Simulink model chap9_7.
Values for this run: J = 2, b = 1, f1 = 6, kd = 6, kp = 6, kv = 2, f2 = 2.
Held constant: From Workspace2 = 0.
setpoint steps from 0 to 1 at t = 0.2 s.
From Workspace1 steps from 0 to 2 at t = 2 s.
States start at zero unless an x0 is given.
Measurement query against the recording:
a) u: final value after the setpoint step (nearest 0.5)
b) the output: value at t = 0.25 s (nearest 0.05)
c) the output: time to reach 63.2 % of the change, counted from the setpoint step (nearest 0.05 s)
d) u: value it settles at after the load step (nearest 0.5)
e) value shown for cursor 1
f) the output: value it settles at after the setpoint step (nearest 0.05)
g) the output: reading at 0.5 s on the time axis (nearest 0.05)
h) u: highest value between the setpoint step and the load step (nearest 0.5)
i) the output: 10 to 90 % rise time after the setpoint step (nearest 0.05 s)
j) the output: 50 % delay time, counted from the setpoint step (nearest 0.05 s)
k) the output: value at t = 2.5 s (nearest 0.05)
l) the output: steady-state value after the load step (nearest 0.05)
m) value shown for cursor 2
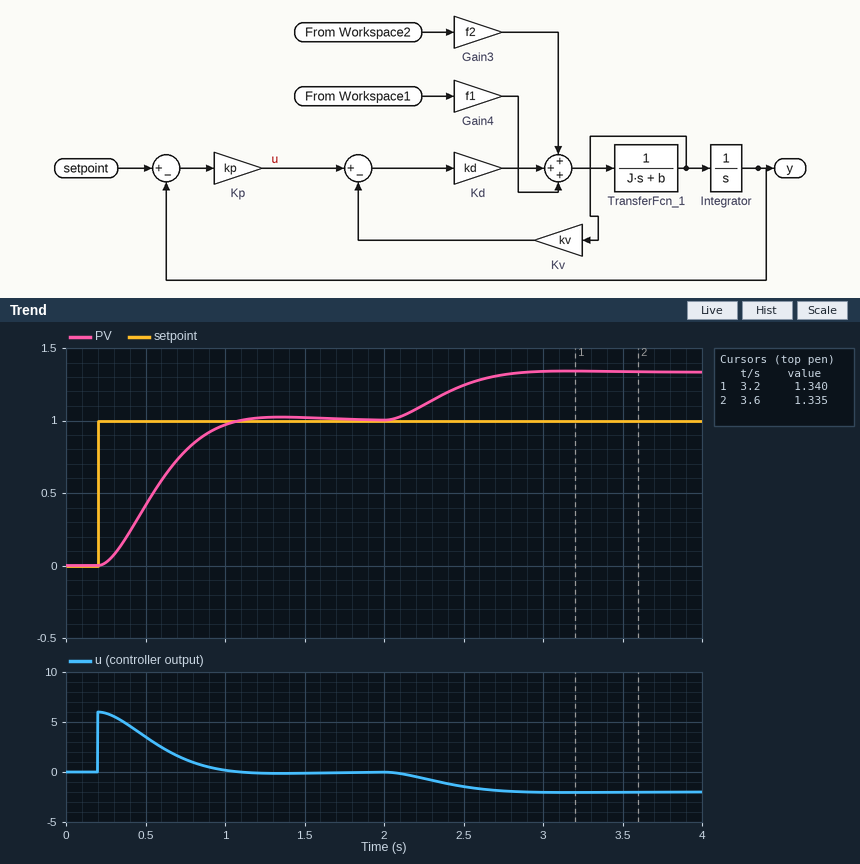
0.0
0.00
0.45 s
-2.0
1.340
1.00
0.40
6.0
0.55 s
0.35 s
1.25
1.35
1.335
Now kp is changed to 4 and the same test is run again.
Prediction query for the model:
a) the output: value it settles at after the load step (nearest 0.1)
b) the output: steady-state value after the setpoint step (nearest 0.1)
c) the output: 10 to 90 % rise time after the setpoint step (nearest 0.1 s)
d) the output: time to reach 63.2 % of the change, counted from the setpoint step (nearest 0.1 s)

1.5
1.0
0.9 s
0.6 s
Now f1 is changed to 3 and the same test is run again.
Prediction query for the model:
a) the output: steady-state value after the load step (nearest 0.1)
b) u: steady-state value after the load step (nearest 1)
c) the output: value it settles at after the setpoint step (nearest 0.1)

1.2
-1
1.0
